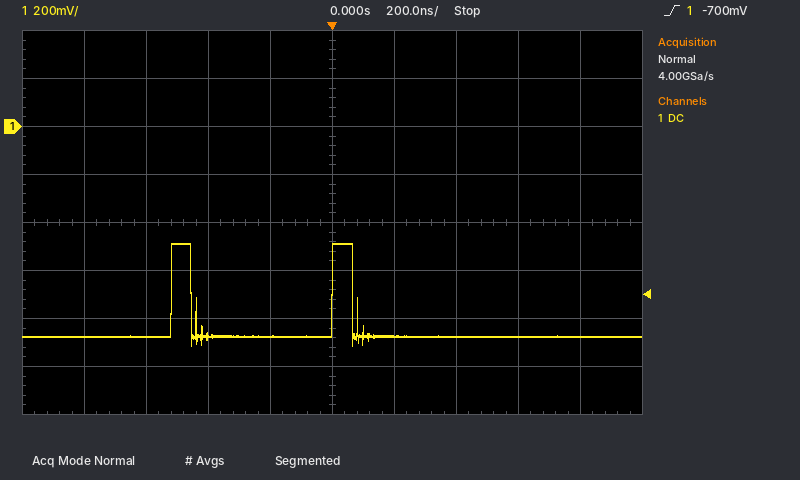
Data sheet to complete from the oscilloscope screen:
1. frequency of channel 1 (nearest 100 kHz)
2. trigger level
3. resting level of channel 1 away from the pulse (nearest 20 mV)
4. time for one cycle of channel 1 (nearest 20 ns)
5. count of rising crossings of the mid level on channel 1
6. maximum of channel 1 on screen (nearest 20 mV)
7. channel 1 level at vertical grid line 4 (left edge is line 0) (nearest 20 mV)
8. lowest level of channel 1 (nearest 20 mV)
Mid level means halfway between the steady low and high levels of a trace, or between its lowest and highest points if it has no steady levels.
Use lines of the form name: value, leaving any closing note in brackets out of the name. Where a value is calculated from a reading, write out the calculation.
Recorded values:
frequency of channel 1: 1 / 520 ns ≈ 1.9 MHz
trigger level: -700 mV
resting level of channel 1 away from the pulse: -880 mV
time for one cycle of channel 1: 520 ns
count of rising crossings of the mid level on channel 1: 2
maximum of channel 1 on screen: -480 mV
channel 1 level at vertical grid line 4 (left edge is line 0): -880 mV
lowest level of channel 1: -920 mV
